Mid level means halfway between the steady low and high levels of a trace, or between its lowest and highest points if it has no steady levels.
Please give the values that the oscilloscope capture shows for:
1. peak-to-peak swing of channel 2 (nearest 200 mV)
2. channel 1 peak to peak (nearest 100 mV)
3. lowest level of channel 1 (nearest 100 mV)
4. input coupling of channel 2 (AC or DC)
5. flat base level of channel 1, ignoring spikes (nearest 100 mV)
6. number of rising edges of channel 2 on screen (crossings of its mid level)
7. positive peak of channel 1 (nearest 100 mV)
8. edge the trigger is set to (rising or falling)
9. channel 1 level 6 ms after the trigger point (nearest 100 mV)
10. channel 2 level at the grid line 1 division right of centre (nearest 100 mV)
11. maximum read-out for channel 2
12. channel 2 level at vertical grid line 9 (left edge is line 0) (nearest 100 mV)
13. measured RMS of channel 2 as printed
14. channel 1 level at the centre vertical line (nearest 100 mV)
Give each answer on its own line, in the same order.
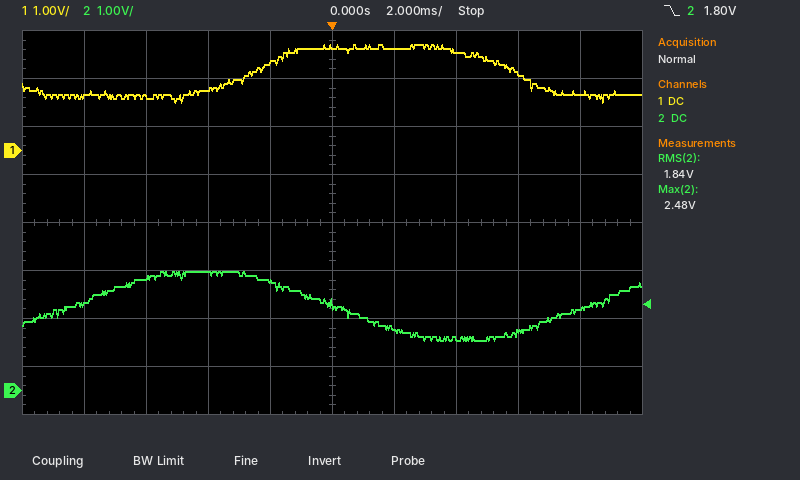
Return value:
1.4 V
1.2 V
1.0 V
DC
1.2 V
2
2.2 V
falling
1.6 V
1.3 V
2.48 V
1.7 V
1.84 V
2.2 V
